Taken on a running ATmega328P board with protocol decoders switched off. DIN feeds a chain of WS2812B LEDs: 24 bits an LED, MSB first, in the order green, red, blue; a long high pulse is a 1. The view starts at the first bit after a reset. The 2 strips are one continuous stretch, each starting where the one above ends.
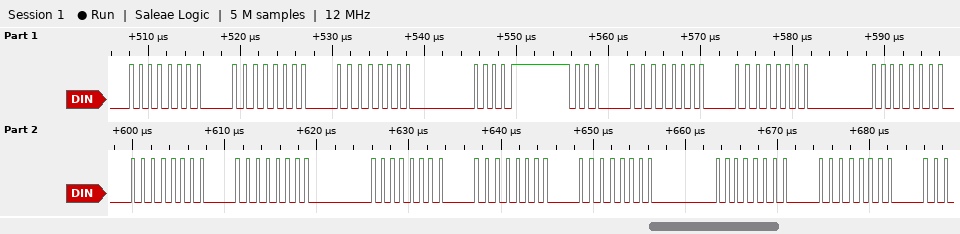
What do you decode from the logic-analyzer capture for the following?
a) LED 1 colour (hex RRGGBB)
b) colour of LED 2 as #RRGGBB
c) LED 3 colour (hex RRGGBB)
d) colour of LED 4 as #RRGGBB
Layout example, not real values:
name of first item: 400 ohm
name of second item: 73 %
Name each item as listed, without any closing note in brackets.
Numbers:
LED 1 colour: #000000
colour of LED 2 as #RRGGBB: #000800
LED 3 colour: #000000
colour of LED 4 as #RRGGBB: #000000
